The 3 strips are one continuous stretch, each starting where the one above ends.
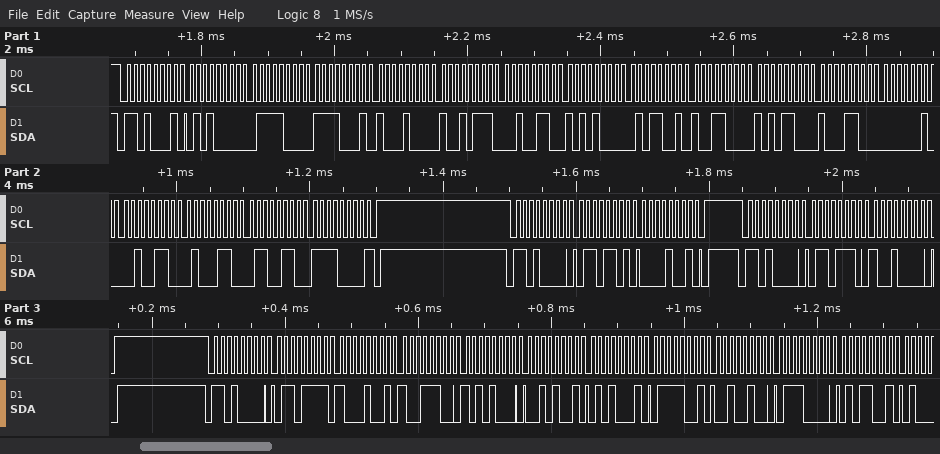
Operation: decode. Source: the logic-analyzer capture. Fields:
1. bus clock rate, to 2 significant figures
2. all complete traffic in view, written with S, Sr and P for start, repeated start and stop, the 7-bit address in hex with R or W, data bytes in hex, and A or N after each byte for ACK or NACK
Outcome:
100 kHz
S 68R A 50 A 78 A F1 A 88 A 97 A 26 A A8 A 59 A 98 A AC A 8C A 02 A 26 A 46 A 66 A F0 N P S 68W A 6D A 09 A P S 68W A 6E A 90 A P S 68W A 6F A 89 A 9C A A8 A 29 A 51 A 79 A 24 A 70 A 59 A
